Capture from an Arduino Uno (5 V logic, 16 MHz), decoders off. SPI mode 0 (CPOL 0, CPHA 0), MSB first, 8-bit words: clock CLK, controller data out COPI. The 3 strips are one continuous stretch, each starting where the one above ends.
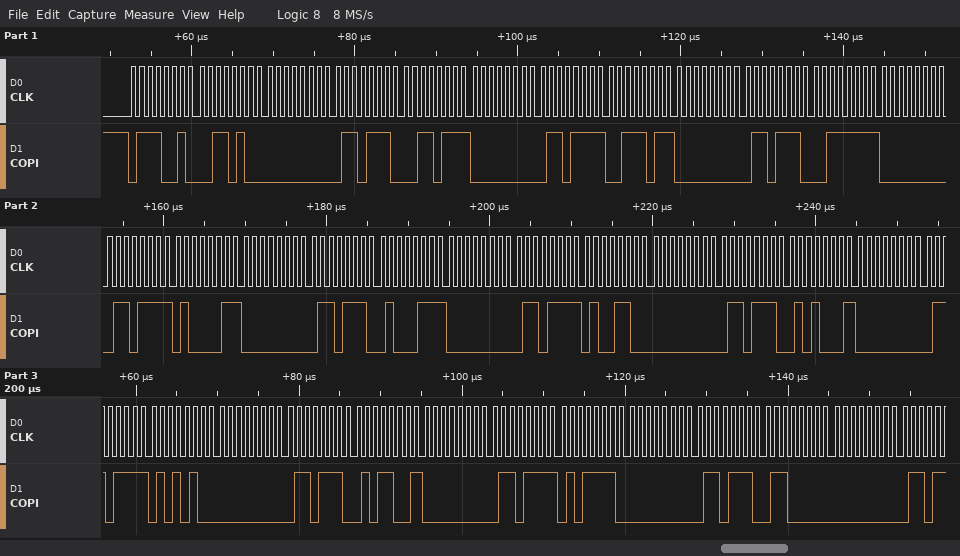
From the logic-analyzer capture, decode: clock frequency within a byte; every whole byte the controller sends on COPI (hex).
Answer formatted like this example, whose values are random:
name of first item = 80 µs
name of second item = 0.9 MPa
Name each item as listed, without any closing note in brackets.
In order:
clock frequency within a byte = 1 MHz
every whole byte the controller sends on COPI = 0x72 0x34 0x00 0x6E 0x37 0x00 0x6F 0x3B 0x00 0x6E 0x3F 0x00 0x6F 0x43 0x00 0x6E 0x47 0x00 0x6F 0x4C 0x00 0x6E 0x51 0x00 0x6F 0x54 0x00 0x6E 0x59 0x00 0x6F 0x5E 0x00 0x6E 0x60 0x00
